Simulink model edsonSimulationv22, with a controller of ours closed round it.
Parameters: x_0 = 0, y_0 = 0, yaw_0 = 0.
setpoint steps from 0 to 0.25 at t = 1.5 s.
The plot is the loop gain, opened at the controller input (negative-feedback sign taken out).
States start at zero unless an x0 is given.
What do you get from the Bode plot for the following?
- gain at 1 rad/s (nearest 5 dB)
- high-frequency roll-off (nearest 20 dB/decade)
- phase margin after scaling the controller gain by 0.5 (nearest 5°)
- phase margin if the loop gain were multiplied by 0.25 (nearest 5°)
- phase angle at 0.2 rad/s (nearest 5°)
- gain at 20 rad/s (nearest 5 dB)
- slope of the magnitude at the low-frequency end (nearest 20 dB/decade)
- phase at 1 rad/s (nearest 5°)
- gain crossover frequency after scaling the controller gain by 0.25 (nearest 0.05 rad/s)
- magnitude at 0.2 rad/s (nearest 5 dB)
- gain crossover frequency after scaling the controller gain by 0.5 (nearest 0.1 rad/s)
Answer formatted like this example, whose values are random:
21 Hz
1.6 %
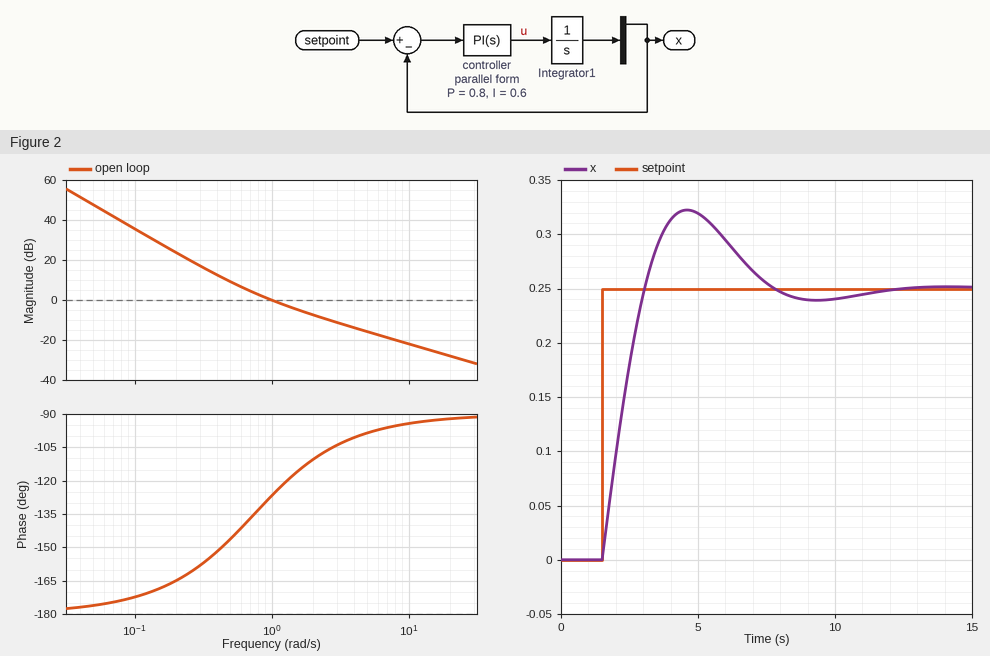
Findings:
0 dB
-20 dB/decade
40°
30°
-165°
-30 dB
-40 dB/decade
-125°
0.40 rad/s
25 dB
0.6 rad/s
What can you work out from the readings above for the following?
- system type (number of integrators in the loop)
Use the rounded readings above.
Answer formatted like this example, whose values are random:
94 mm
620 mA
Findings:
2
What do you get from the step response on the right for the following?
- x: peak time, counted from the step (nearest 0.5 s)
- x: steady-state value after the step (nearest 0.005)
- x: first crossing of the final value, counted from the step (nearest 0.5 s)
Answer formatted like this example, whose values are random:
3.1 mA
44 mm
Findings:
3.0 s
0.250
1.5 s
